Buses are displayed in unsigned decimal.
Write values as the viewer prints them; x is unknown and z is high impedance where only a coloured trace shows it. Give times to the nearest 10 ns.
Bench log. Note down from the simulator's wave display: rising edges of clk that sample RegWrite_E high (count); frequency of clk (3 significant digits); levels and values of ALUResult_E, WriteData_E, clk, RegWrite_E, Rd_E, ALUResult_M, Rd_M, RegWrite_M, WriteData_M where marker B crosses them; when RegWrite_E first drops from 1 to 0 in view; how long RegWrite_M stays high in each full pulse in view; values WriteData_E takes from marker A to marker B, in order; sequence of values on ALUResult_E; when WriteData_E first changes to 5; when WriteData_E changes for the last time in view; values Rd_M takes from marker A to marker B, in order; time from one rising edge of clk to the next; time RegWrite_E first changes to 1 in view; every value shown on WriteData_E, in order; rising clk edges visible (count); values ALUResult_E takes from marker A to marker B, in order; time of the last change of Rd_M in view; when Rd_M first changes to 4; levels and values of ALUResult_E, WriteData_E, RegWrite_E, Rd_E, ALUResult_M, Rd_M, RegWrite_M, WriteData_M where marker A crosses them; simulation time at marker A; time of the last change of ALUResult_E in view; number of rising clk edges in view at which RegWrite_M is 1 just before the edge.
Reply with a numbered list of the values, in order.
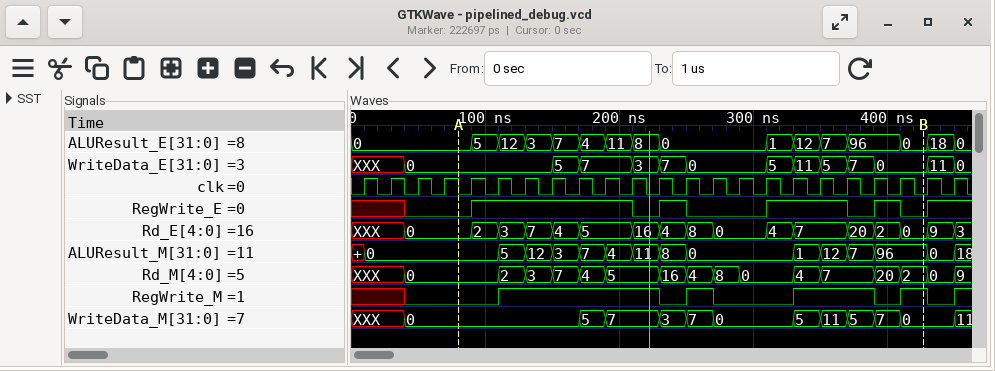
1. 12
2. 50.0 MHz
3. ALUResult_E=0, WriteData_E=0, clk=0, RegWrite_E=0, Rd_E=0, ALUResult_M=96, Rd_M=2, RegWrite_M=1, WriteData_M=0
4. 210 ns
5. 120 ns, 20 ns, 60 ns, 20 ns
6. 0, 5, 7, 3, 7, 0, 5, 11, 5, 7, 0
7. 0, 5, 12, 3, 7, 4, 11, 8, 0, 1, 12, 7, 96, 0, 18, 0
8. 150 ns
9. 450 ns
10. 0, 2, 3, 7, 4, 5, 16, 4, 8, 0, 4, 7, 20, 2
11. 20 ns
12. 90 ns
13. XXX, 0, 5, 7, 3, 7, 0, 5, 11, 5, 7, 0, 11, 0
14. 23
15. 0, 5, 12, 3, 7, 4, 11, 8, 0, 1, 12, 7, 96, 0
16. 450 ns
17. 170 ns
18. ALUResult_E=0, WriteData_E=0, RegWrite_E=0, Rd_E=0, ALUResult_M=0, Rd_M=0, RegWrite_M=0, WriteData_M=0
19. 80 ns
20. 450 ns
21. 11
